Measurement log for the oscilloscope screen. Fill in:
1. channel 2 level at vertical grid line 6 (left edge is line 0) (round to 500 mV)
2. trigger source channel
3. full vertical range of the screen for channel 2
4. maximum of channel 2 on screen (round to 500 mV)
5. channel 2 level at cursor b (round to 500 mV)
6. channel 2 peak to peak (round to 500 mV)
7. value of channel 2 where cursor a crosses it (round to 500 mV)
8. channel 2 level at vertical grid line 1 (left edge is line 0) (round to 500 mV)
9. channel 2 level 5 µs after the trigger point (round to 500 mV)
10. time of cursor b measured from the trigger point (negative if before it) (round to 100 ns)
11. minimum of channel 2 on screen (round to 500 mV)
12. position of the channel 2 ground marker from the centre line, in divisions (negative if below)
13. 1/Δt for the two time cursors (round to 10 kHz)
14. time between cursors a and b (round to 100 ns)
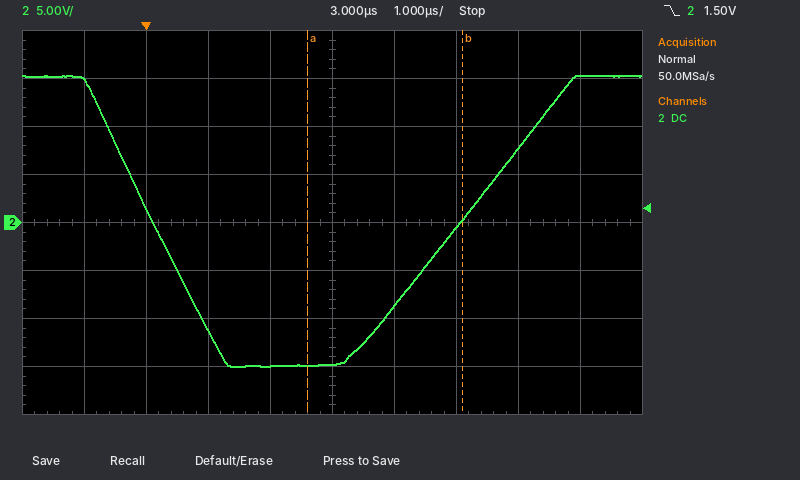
-8.5 V
channel 2
40 V
15.5 V
500 mV
30.5 V
-15.0 V
15.0 V
-500 mV
+5.1 µs
-15.0 V
0.0 div
400 kHz
2.5 µs
